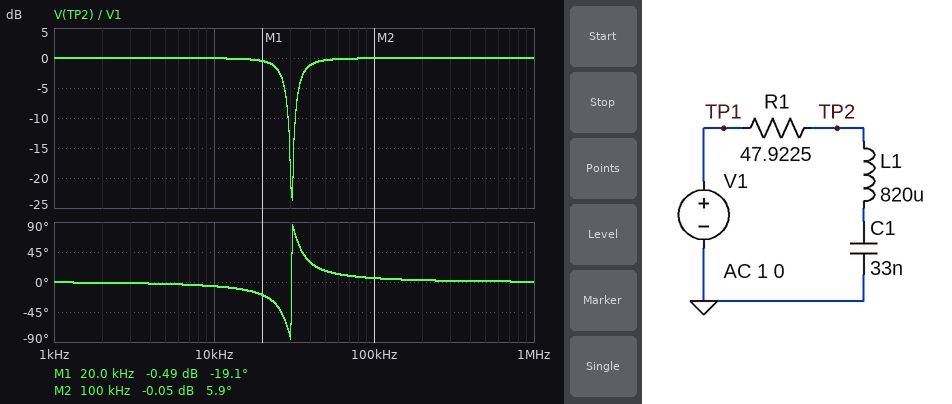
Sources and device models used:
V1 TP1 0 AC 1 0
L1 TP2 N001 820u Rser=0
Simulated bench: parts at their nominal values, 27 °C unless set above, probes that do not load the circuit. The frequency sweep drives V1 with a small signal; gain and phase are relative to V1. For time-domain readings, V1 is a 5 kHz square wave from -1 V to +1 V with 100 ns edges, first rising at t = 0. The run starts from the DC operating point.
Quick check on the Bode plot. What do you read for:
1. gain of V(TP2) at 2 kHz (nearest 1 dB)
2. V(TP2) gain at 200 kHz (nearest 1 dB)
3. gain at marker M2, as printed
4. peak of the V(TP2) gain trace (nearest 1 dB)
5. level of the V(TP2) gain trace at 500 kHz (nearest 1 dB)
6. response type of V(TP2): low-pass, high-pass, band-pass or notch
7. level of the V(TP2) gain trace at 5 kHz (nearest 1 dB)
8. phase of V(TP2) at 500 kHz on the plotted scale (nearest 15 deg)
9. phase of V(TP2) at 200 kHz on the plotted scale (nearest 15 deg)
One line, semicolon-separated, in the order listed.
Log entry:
0 dB; 0 dB; -0.05 dB; 0 dB; 0 dB; notch; 0 dB; 0 deg; 0 deg
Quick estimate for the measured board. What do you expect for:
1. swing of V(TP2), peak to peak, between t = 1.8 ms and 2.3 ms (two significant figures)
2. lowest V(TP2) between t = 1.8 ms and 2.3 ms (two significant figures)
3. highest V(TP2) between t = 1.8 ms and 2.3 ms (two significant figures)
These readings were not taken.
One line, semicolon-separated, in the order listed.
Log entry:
2.6 V; -1.3 V; 1.3 V
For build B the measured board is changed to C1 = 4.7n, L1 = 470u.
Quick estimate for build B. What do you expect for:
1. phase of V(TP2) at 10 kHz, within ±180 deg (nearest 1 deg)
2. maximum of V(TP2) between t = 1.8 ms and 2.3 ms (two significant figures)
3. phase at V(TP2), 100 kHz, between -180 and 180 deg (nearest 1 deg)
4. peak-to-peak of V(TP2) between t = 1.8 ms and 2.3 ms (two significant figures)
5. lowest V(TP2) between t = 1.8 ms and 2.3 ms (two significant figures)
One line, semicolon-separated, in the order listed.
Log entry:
-1 deg; 1.2 V; -48 deg; 2.4 V; -1.2 V
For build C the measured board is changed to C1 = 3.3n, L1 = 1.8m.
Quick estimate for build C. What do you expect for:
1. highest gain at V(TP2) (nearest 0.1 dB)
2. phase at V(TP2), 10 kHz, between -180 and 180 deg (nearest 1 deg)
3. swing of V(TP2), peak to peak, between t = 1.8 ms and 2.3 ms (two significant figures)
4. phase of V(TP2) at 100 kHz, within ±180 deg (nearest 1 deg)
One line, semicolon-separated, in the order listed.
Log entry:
0 dB; -1 deg; 2.3 V; 4 deg
